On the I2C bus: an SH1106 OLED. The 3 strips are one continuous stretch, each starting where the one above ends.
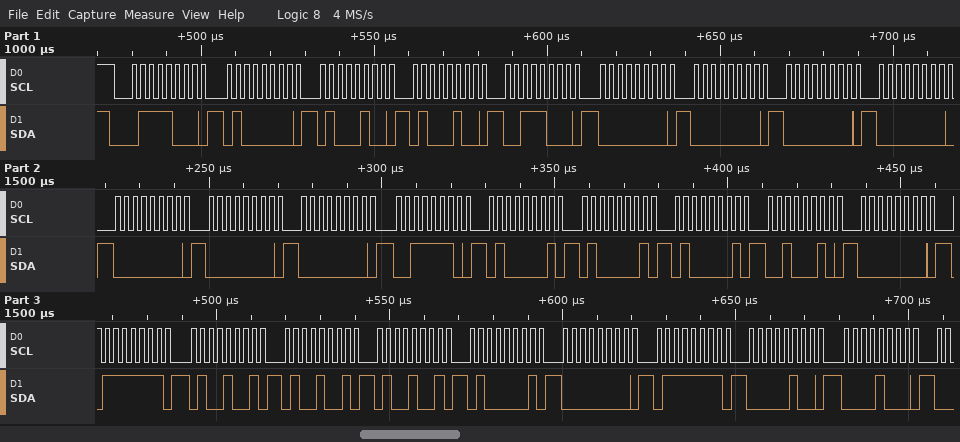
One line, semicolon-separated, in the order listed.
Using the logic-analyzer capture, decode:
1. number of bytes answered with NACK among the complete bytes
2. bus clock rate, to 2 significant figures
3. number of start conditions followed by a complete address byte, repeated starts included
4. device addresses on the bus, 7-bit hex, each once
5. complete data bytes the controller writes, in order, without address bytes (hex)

0; 400 kHz; 1; 0x3C; 40 44 44 38 00 00 00 00 00 00 00 3E 41 41 41 22 00 7F 49 49 49 41 00 7F 04 08
